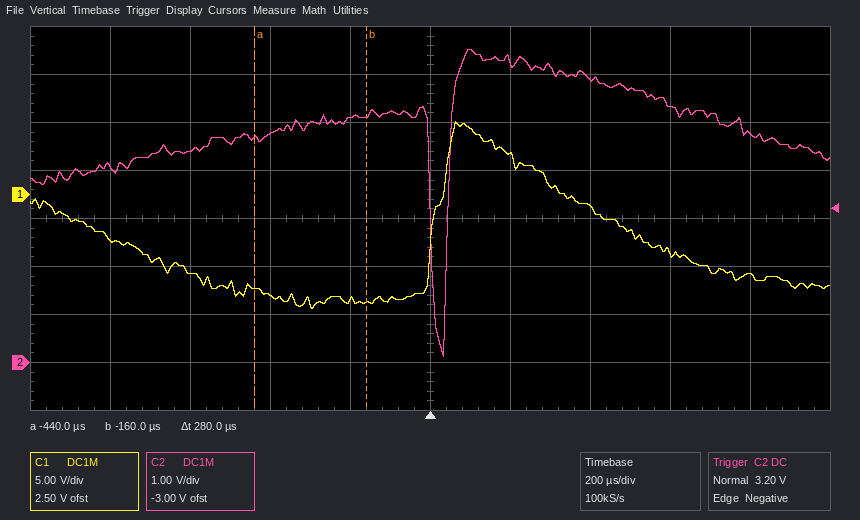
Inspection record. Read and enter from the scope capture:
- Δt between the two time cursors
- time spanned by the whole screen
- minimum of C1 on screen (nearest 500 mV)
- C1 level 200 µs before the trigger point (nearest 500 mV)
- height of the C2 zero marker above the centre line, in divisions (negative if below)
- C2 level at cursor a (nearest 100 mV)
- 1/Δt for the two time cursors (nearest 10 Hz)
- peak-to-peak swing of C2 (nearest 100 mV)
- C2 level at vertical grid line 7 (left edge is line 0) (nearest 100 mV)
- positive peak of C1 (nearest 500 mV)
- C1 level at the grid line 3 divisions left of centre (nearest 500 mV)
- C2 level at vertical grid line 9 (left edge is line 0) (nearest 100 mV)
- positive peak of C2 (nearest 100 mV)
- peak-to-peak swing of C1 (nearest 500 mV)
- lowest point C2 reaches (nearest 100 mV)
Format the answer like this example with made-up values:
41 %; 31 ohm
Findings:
280 µs; 2 ms; -12.0 V; -11.0 V; -3.0 div; 4.7 V; 3.57 kHz; 6.4 V; 5.9 V; 7.5 V; -8.0 V; 4.8 V; 6.5 V; 19.5 V; 100 mV
